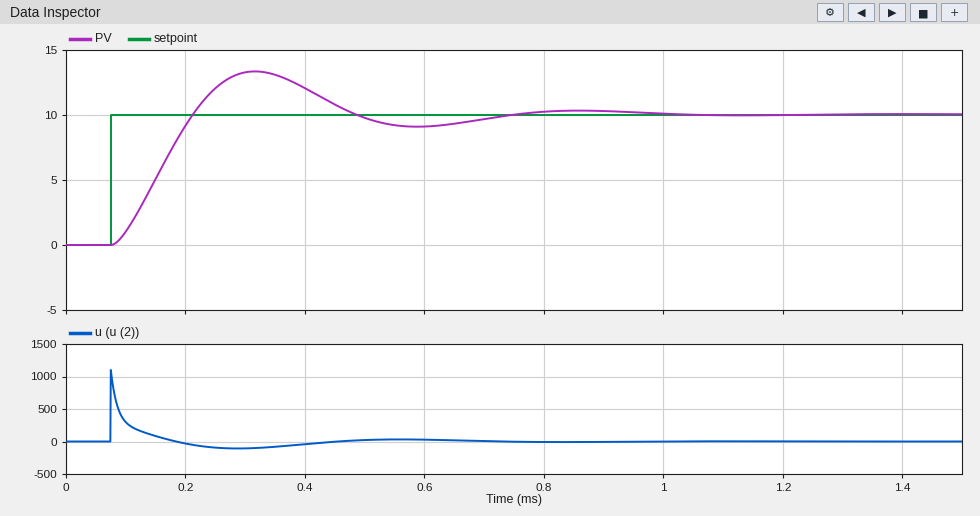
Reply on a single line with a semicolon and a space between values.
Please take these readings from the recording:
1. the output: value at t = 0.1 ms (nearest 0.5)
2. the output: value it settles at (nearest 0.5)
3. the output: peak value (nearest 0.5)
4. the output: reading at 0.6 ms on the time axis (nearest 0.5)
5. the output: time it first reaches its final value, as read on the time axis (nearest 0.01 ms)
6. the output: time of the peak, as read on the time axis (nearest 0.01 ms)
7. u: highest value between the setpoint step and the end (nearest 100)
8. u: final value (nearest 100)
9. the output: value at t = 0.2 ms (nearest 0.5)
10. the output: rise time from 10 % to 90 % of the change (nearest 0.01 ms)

1.0; 10.0; 13.5; 9.0; 0.21 ms; 0.32 ms; 1100; 0; 9.0; 0.10 ms
